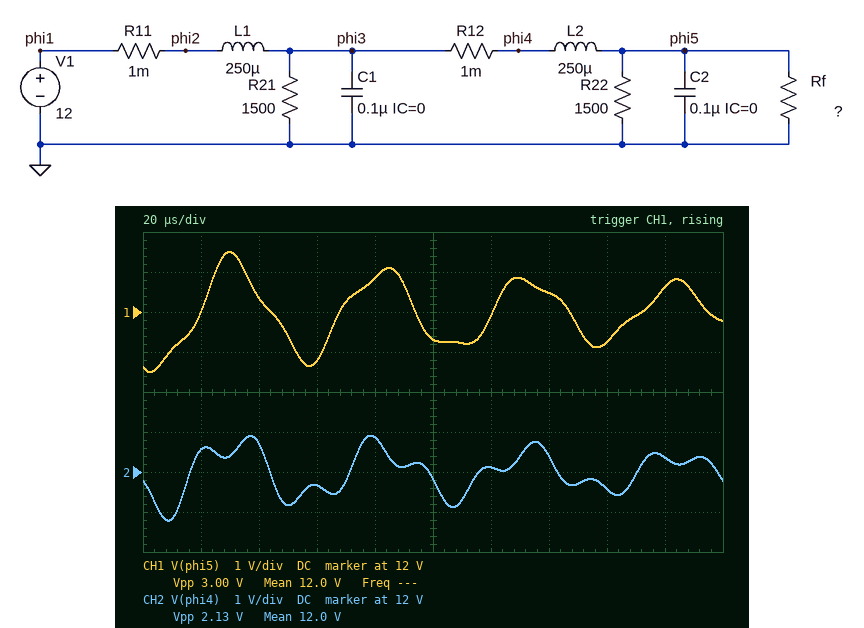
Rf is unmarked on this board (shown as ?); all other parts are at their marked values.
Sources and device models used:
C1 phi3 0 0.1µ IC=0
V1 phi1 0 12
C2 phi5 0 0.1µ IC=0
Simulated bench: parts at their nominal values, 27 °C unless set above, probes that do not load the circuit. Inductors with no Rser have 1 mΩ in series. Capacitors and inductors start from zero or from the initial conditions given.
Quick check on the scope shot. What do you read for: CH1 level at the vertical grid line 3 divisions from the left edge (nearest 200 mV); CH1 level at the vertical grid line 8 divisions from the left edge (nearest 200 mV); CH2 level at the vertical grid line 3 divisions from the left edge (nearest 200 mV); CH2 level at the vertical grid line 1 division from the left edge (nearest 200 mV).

10.8 V
11.2 V
11.6 V
12.6 V
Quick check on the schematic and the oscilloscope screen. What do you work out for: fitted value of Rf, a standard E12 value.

4.7 kΩ
